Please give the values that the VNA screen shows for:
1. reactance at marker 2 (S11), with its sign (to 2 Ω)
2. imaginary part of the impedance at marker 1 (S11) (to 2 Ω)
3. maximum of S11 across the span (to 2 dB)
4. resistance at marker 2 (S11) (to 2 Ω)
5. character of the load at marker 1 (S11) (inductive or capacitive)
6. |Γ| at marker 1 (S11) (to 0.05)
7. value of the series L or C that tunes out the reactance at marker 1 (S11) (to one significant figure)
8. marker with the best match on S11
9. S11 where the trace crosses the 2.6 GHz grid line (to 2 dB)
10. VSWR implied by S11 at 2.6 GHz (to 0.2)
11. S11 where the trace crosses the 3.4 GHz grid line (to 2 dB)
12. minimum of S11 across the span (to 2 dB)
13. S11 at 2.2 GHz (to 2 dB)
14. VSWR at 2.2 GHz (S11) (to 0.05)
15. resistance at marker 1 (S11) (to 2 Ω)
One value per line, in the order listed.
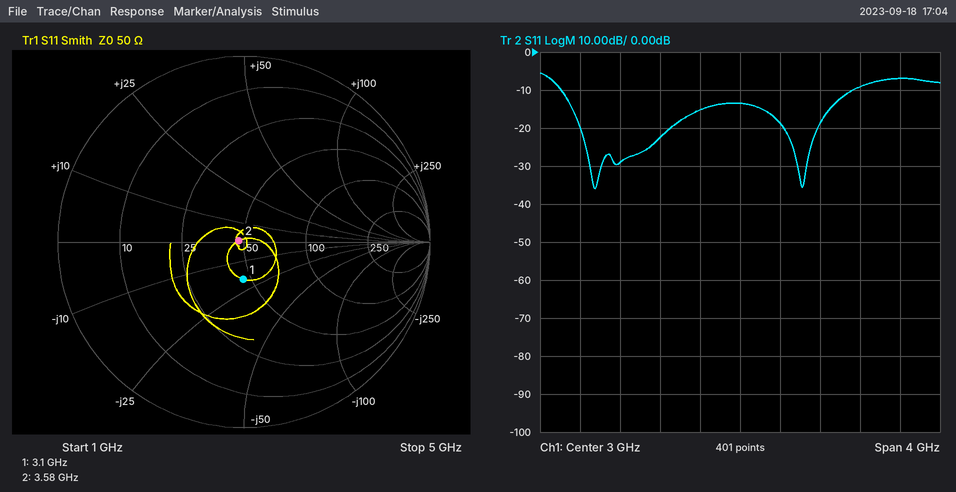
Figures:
0 Ω
-20 Ω
-6 dB
48 Ω
capacitive
0.20
1.0 nH
marker 2
-16 dB
1.4
-18 dB
-36 dB
-22 dB
1.15
46 Ω
